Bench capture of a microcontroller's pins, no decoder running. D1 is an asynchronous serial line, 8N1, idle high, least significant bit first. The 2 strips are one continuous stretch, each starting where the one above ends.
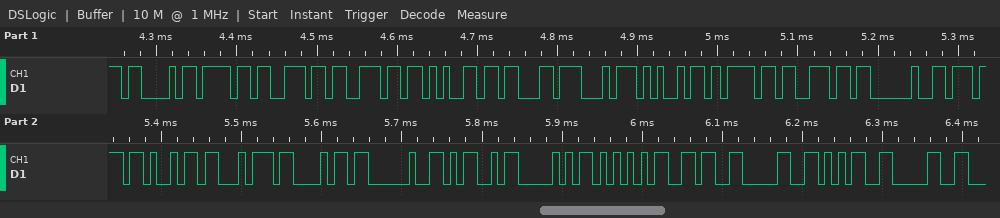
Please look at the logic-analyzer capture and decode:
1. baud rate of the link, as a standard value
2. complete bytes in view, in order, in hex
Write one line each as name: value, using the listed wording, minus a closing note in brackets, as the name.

baud rate of the link, as a standard value: 115200 baud
complete bytes in view, in order, in hex: 43 6F 6E 6E 65 63 74 69 6F 6E 20 77 69 74 68 20 4D 50 55 36 30 35 30
